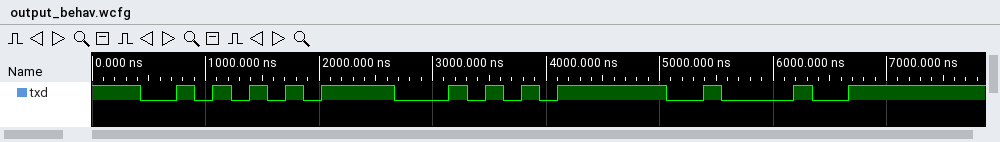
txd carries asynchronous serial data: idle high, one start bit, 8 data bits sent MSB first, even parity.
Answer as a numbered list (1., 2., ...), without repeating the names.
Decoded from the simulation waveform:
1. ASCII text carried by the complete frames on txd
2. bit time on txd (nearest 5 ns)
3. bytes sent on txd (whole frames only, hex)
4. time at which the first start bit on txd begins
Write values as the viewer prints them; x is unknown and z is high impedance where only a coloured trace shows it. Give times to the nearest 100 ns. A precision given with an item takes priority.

1. "U*B"
2. 160 ns
3. 55, 2A, 42
4. 400 ns
